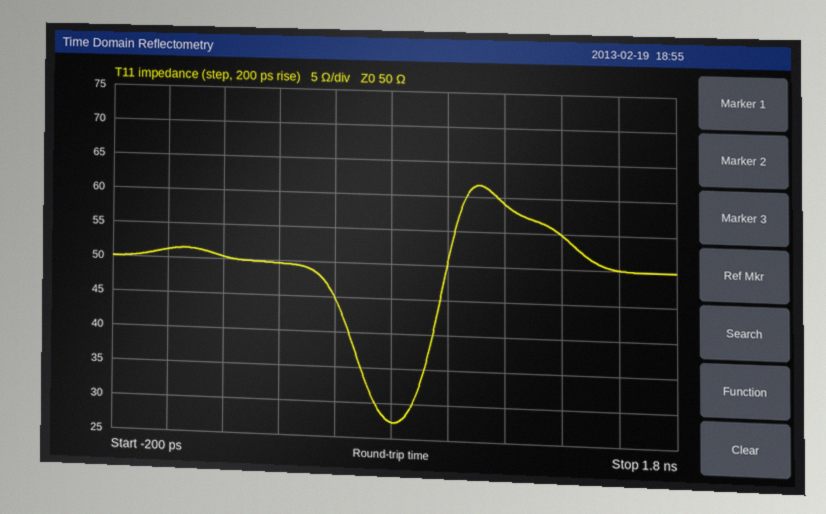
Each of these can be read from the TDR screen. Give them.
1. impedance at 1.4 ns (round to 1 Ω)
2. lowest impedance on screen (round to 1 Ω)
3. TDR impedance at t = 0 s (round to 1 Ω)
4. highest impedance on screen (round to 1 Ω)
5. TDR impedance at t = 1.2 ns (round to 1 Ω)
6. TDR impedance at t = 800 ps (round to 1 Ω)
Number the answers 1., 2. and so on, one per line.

1. 55 Ω
2. 27 Ω
3. 51 Ω
4. 62 Ω
5. 59 Ω
6. 27 Ω
